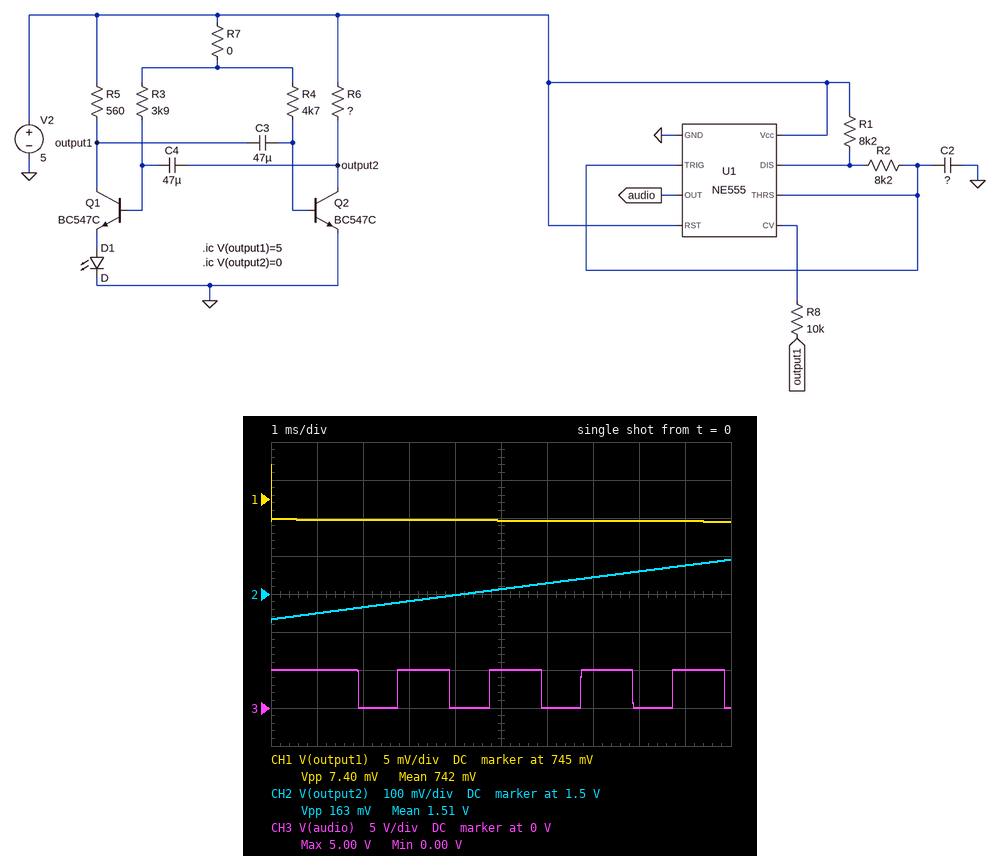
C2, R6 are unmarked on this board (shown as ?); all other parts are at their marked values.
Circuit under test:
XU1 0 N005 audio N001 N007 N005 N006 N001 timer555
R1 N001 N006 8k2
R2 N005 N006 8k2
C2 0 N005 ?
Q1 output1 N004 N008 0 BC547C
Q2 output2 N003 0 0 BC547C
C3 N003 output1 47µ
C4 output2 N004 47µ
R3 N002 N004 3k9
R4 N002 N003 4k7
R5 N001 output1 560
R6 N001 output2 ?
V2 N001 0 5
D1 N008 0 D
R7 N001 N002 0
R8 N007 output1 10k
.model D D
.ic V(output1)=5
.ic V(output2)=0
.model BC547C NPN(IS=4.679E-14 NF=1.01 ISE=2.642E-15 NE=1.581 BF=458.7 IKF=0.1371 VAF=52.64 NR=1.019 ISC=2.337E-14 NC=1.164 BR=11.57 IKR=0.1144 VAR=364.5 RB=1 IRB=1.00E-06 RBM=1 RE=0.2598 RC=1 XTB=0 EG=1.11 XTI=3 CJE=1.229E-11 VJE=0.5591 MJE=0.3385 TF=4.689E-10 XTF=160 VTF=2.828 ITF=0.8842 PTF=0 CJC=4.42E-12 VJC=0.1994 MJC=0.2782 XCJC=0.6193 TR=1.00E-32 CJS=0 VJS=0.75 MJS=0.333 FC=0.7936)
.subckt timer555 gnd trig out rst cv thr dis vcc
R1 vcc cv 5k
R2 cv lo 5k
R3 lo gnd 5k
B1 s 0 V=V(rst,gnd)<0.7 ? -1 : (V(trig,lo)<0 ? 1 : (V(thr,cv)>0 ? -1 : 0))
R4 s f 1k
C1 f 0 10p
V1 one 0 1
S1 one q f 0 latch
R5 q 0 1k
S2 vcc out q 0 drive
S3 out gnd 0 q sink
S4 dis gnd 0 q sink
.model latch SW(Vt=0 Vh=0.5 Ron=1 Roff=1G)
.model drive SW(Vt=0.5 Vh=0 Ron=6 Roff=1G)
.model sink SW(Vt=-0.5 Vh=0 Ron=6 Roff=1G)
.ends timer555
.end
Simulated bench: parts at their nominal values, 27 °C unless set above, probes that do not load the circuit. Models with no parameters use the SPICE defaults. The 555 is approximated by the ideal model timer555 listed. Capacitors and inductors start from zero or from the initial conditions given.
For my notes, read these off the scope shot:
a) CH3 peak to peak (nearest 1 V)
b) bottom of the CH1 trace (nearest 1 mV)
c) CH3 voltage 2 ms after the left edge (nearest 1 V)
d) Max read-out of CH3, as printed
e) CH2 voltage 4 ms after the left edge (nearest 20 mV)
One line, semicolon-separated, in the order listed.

5 V; 742 mV; 0 V; 5.00 V; 1.50 V
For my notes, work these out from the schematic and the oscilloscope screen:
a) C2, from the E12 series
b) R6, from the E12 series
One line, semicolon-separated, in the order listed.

150 nF; 4.7 kΩ
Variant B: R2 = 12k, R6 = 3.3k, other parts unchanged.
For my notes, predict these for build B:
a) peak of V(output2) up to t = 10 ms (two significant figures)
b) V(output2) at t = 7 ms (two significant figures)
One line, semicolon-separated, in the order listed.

1.7 V; 1.6 V
